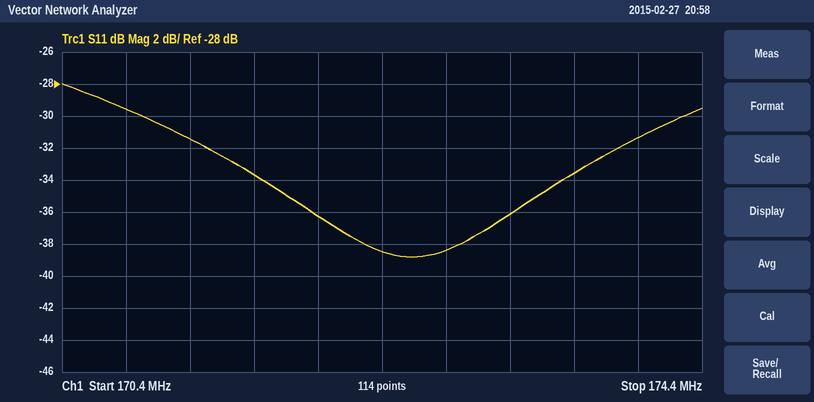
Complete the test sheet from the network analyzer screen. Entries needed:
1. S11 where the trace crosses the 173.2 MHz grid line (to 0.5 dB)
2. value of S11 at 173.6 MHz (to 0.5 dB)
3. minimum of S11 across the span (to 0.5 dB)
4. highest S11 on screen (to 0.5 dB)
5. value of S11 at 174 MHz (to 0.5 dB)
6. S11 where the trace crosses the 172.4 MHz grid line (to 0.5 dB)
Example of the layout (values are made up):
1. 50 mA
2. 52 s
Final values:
1. -36.0 dB
2. -33.5 dB
3. -39.0 dB
4. -28.0 dB
5. -31.5 dB
6. -38.5 dB
